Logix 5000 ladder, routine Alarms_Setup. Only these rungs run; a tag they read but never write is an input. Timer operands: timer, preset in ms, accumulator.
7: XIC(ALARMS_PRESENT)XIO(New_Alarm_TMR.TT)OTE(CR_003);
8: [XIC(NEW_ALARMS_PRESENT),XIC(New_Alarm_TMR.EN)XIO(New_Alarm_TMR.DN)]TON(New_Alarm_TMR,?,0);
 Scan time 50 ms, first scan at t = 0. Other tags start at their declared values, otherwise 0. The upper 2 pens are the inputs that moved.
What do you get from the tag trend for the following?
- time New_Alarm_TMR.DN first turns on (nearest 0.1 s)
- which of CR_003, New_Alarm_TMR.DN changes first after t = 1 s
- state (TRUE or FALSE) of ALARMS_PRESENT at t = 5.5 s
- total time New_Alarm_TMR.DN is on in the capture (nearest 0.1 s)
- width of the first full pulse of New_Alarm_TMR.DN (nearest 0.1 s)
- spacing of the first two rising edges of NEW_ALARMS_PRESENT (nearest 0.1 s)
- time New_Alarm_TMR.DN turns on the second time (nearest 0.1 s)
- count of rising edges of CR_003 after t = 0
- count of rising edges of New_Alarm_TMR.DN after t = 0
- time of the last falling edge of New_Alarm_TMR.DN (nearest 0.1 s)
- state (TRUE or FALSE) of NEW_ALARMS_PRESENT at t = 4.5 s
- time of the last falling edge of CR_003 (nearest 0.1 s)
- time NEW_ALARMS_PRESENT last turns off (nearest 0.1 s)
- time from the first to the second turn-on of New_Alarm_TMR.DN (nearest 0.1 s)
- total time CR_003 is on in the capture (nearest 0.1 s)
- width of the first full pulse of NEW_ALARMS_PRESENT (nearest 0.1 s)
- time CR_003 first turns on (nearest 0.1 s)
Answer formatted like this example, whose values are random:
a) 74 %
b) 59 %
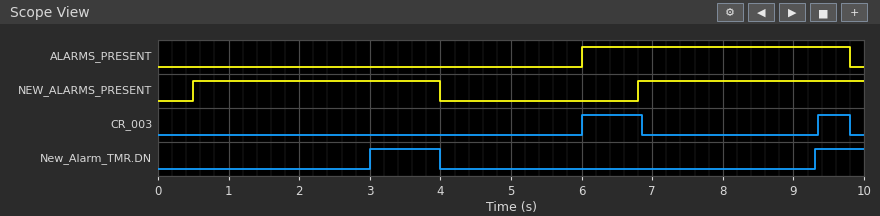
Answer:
a) 3.0 s
b) New_Alarm_TMR.DN
c) FALSE
d) 1.7 s
e) 1.0 s
f) 6.3 s
g) 9.3 s
h) 2
i) 2
j) 4.0 s
k) FALSE
l) 9.8 s
m) 4.0 s
n) 6.3 s
o) 1.3 s
p) 3.5 s
q) 6.0 s
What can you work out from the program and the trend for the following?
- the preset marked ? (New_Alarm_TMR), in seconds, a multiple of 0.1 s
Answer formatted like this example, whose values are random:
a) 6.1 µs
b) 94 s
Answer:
a) 2.5 s
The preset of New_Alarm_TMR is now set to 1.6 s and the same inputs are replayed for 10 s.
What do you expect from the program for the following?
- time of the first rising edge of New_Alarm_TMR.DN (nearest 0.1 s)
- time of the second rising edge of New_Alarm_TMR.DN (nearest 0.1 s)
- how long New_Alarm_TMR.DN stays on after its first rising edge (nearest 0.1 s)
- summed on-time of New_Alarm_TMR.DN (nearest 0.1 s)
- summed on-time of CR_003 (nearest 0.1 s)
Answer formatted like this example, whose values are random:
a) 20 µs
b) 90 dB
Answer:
a) 2.1 s
b) 8.4 s
c) 1.9 s
d) 3.5 s
e) 2.2 s
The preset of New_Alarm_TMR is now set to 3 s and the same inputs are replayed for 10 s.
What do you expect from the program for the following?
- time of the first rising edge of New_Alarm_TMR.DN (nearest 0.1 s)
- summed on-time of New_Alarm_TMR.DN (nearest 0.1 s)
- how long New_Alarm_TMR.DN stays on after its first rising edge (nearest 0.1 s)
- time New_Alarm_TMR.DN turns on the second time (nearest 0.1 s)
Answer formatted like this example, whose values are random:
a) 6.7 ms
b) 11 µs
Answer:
a) 3.5 s
b) 0.7 s
c) 0.5 s
d) 9.8 s
